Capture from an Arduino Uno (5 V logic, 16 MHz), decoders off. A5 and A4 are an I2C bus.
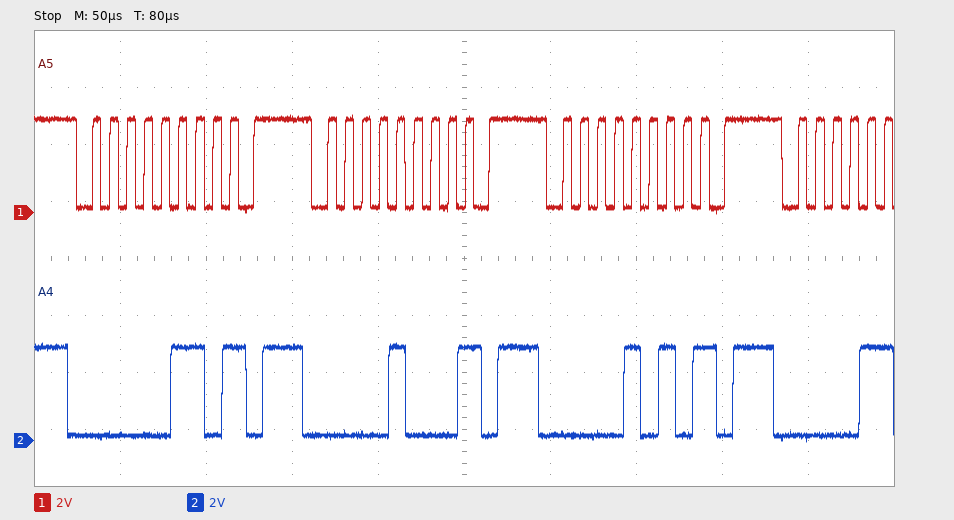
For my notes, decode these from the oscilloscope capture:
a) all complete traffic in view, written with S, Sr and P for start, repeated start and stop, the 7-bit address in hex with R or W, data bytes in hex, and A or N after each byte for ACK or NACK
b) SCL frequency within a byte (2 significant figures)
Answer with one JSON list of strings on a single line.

["S 03W N P S 04W N P S 05W N P", "100 kHz"]
